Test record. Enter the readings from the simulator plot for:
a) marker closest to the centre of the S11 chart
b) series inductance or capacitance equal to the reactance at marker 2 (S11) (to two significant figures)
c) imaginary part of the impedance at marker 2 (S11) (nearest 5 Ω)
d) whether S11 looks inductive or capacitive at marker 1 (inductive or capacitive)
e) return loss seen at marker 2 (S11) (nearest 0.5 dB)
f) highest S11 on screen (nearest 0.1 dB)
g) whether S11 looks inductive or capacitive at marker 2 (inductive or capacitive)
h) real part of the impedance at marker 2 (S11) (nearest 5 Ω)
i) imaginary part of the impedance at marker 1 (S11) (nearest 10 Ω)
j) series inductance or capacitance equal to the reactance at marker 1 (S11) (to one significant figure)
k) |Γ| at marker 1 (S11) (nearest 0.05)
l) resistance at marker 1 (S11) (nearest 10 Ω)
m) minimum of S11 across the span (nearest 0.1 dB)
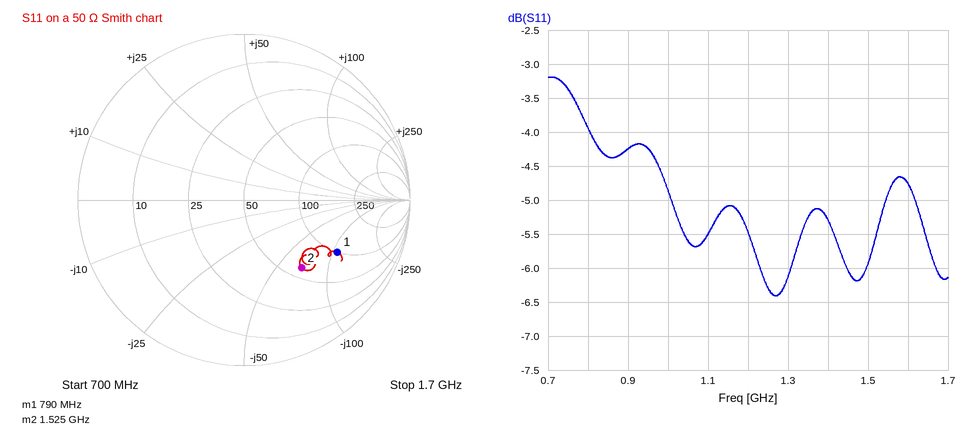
marker 2
1.5 pF
-70 Ω
capacitive
5.5 dB
-3.2 dB
capacitive
60 Ω
-110 Ω
2 pF
0.65
100 Ω
-6.4 dB
